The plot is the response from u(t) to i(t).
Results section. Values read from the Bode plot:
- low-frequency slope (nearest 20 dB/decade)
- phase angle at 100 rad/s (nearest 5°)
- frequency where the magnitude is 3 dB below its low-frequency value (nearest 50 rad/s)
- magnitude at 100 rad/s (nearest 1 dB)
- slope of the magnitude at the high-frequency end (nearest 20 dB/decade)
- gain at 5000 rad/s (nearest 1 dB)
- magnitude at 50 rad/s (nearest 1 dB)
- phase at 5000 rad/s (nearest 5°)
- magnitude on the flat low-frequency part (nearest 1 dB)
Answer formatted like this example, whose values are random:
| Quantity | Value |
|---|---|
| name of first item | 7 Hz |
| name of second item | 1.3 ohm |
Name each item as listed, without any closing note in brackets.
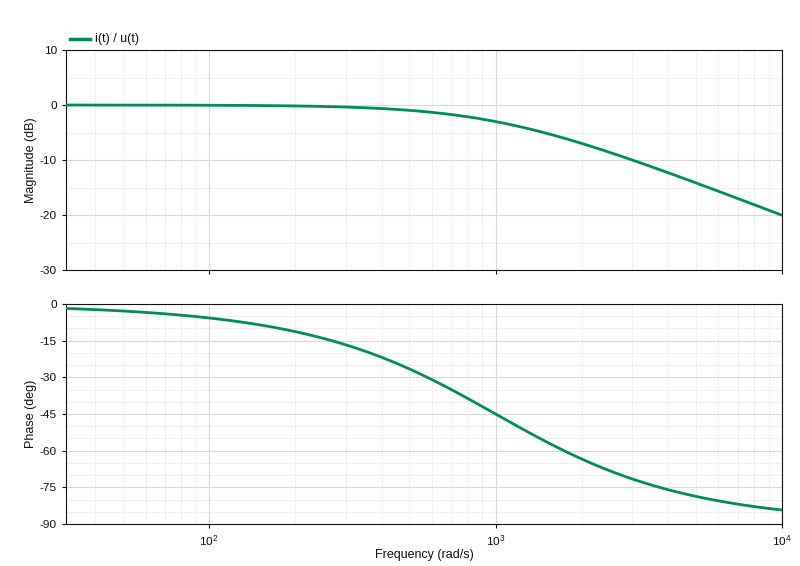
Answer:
| Quantity | Value |
|---|---|
| low-frequency slope | 0 dB/decade |
| phase angle at 100 rad/s | -5° |
| frequency where the magnitude is 3 dB below its low-frequency value | 1000 rad/s |
| magnitude at 100 rad/s | 0 dB |
| slope of the magnitude at the high-frequency end | -20 dB/decade |
| gain at 5000 rad/s | -14 dB |
| magnitude at 50 rad/s | 0 dB |
| phase at 5000 rad/s | -80° |
| magnitude on the flat low-frequency part | 0 dB |
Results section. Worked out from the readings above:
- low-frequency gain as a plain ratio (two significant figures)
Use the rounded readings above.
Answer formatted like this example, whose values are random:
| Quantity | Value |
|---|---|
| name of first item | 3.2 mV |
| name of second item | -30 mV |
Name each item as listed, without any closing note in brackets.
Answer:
| Quantity | Value |
|---|---|
| low-frequency gain as a plain ratio | 1.0 |
